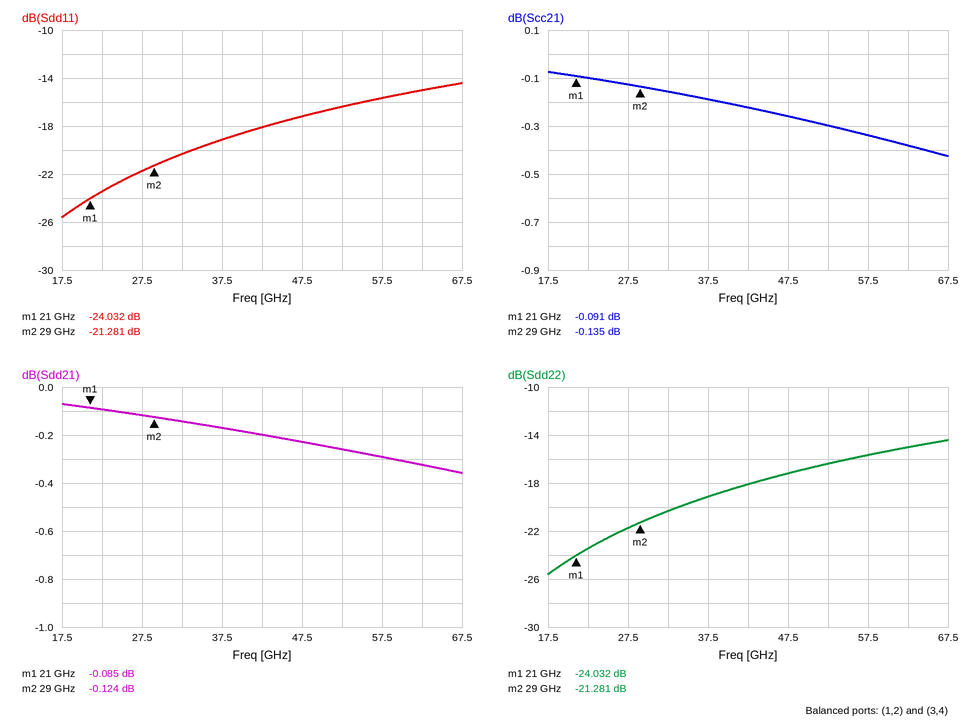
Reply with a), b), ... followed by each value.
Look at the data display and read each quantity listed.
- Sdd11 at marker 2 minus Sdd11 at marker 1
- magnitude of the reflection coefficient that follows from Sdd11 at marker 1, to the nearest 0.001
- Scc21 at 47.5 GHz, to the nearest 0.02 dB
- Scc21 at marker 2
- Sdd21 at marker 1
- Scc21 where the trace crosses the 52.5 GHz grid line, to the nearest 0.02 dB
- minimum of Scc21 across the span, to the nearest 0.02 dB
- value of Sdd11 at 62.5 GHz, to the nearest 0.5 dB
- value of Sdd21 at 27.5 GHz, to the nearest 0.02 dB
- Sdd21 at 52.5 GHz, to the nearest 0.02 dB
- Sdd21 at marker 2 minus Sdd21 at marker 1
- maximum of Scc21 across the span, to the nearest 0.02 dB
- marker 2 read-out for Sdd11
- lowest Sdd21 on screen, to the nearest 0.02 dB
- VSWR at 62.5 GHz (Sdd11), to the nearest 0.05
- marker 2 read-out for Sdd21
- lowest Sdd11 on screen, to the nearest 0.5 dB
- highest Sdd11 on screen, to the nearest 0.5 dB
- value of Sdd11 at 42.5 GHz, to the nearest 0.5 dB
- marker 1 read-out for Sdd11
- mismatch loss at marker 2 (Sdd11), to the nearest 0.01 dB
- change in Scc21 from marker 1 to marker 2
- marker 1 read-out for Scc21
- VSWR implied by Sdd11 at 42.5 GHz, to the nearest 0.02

a) 2.751 dB
b) 0.063
c) -0.26 dB
d) -0.135 dB
e) -0.085 dB
f) -0.30 dB
g) -0.42 dB
h) -15.0 dB
i) -0.12 dB
j) -0.26 dB
k) -0.039 dB
l) -0.08 dB
m) -21.281 dB
n) -0.36 dB
o) 1.45
p) -0.124 dB
q) -25.5 dB
r) -14.5 dB
s) -18.0 dB
t) -24.032 dB
u) 0.03 dB
v) -0.044 dB
w) -0.091 dB
x) 1.28
